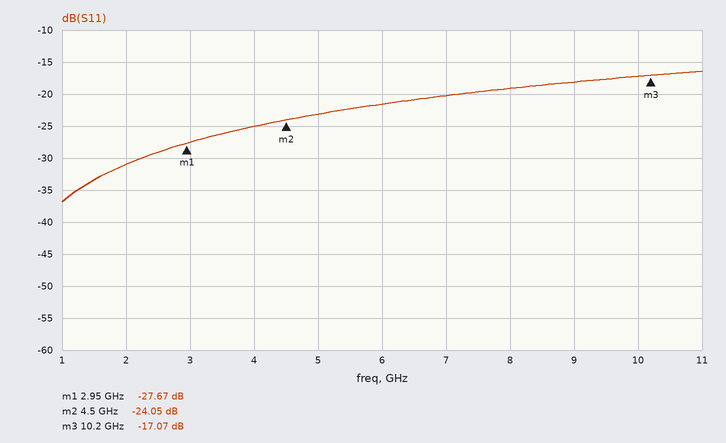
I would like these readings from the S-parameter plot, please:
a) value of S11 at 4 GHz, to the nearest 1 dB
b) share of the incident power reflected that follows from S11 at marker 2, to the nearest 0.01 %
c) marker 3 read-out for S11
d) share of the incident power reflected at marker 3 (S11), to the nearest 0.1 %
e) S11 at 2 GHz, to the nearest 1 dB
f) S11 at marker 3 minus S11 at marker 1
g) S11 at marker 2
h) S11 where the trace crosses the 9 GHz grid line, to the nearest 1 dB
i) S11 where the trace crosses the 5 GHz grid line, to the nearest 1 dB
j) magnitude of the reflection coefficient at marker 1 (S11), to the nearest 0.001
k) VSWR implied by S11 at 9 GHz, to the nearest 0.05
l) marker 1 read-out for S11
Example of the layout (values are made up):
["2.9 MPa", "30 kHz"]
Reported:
["-25 dB", "0.39 %", "-17.07 dB", "2.0 %", "-31 dB", "10.60 dB", "-24.05 dB", "-18 dB", "-23 dB", "0.041", "1.30", "-27.67 dB"]
